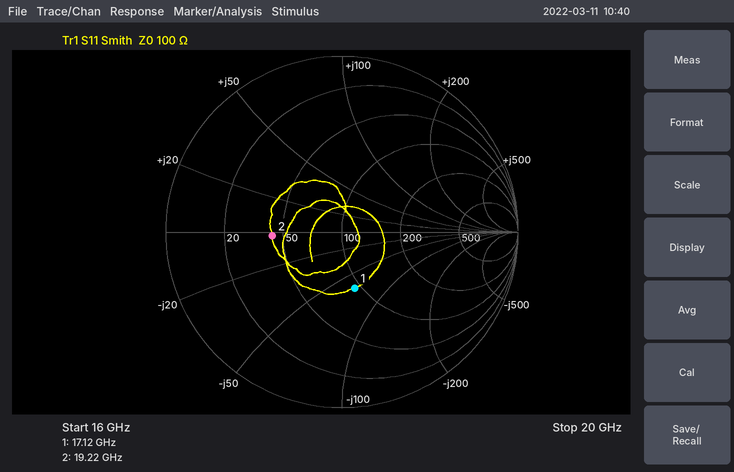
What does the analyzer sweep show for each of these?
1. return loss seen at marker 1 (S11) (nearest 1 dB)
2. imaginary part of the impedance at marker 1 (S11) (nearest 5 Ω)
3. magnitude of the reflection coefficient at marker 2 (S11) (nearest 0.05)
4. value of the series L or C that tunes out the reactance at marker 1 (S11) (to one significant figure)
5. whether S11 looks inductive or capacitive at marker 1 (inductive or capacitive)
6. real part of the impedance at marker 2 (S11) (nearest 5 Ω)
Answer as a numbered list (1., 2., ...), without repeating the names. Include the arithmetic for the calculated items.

1. 10 dB
2. -65 Ω
3. 0.40
4. L = 65 Ω/(2π × 17.12 GHz) ≈ 604 pH, so 600 pH to one significant figure
5. capacitive
6. 45 Ω
